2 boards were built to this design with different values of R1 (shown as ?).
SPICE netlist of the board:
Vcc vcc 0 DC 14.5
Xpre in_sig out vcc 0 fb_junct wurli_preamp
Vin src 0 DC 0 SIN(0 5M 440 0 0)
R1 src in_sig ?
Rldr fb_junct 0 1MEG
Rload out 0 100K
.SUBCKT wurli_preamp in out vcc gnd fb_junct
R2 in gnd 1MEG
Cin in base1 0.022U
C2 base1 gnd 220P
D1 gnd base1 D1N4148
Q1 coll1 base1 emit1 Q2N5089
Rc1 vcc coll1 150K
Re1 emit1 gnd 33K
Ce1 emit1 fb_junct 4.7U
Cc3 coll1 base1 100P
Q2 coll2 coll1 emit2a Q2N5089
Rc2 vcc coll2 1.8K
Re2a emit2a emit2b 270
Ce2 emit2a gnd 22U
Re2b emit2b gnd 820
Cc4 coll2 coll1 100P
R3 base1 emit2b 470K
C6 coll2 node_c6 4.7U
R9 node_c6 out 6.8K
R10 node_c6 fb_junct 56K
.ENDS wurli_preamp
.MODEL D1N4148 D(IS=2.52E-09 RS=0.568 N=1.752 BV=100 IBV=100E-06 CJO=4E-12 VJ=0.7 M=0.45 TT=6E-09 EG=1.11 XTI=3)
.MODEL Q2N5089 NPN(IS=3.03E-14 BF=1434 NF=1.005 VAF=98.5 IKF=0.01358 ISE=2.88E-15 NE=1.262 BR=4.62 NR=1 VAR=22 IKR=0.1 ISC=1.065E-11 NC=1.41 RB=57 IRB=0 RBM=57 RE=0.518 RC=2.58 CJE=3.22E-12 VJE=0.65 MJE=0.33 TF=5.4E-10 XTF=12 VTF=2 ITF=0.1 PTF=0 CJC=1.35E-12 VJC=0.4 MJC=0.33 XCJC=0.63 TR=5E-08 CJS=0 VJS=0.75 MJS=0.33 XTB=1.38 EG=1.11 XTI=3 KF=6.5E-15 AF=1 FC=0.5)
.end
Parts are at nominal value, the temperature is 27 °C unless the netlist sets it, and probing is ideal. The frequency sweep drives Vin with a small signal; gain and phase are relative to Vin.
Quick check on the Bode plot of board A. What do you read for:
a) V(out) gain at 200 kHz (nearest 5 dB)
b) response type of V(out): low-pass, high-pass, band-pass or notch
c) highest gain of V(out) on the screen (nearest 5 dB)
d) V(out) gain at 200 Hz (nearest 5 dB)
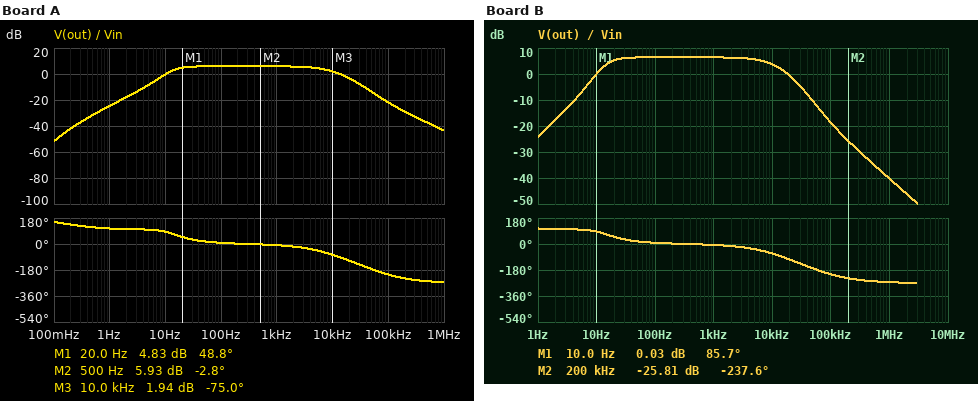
-30 dB
band-pass
5 dB
5 dB
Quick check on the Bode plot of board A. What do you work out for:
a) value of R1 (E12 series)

68 kΩ
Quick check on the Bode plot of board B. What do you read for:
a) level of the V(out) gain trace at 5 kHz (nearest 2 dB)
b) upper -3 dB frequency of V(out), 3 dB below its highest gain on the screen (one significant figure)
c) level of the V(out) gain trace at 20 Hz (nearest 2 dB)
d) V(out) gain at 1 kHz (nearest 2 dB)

6 dB
10 kHz
6 dB
6 dB
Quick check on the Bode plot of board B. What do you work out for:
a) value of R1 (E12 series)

47 kΩ
